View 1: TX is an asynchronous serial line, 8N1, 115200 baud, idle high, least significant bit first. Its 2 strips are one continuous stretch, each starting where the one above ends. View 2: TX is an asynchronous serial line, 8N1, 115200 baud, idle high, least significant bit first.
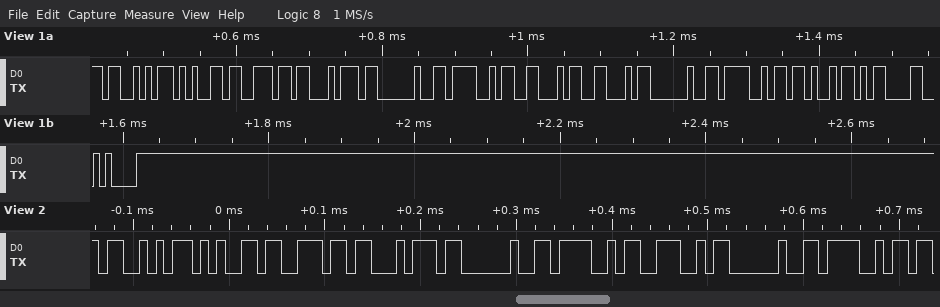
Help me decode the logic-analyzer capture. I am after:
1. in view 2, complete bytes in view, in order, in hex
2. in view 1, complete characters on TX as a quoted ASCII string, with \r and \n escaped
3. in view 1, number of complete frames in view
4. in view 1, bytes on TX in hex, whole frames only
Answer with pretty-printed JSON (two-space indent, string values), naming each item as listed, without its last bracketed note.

{
  "in view 2, complete bytes in view, in order, in hex": "0x53 0x65 0x6E 0x74 0x20 0x4F 0x4E 0x20 0x4F",
  "in view 1, complete characters on TX as a quoted ASCII string, with \\r and \\n escaped": "\"Sent OFF OK\\r\\n\"",
  "in view 1, number of complete frames in view": "13",
  "in view 1, bytes on TX in hex, whole frames only": "0x53 0x65 0x6E 0x74 0x20 0x4F 0x46 0x46 0x20 0x4F 0x4B 0x0D 0x0A"
}
